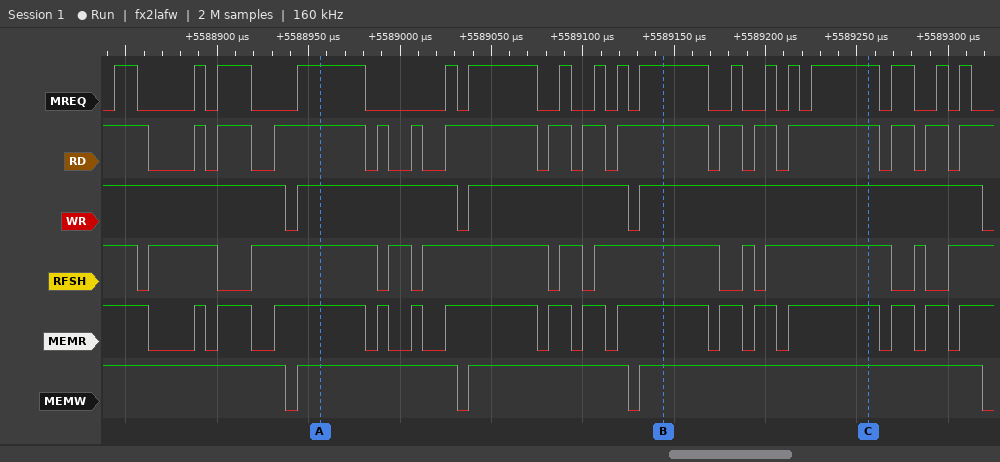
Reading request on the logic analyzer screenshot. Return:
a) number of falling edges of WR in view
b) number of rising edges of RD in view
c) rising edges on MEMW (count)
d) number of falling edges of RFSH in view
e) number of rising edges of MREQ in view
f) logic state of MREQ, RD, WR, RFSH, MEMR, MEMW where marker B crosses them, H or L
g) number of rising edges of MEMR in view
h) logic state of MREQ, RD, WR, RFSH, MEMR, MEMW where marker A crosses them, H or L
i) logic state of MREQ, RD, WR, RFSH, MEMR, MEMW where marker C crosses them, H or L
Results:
4
15
3
10
17
MREQ=H, RD=H, WR=H, RFSH=H, MEMR=H, MEMW=H
15
MREQ=H, RD=H, WR=H, RFSH=H, MEMR=H, MEMW=H
MREQ=H, RD=H, WR=H, RFSH=H, MEMR=H, MEMW=H
